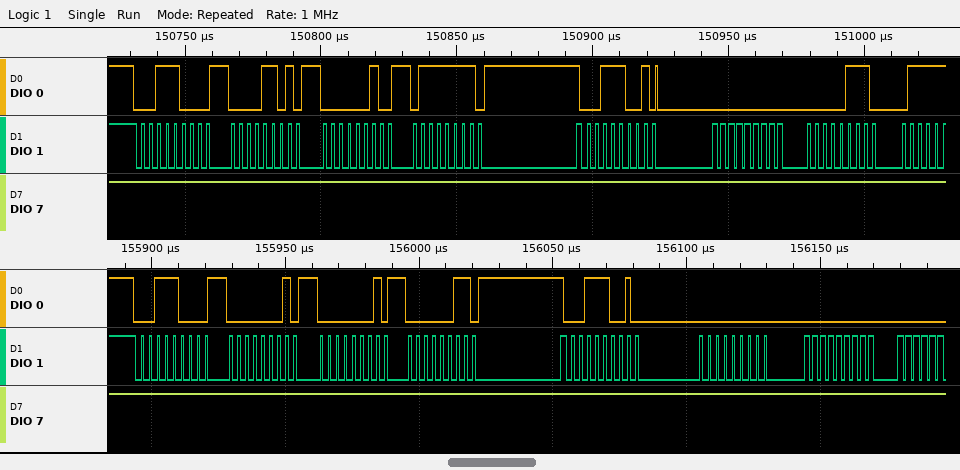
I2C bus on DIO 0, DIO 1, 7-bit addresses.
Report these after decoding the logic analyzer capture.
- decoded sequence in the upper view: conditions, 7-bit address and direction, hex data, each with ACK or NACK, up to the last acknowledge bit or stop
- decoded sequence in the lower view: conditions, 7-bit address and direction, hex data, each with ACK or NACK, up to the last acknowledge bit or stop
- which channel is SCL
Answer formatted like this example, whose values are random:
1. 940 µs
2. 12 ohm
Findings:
1. start, address 1C write ACK, 0D ACK, 02 ACK, 7F ACK, repeated start, address 1C read ACK, 00 ACK, 07 ACK
2. start, address 1C write ACK, 01 ACK, 01 ACK, 03 ACK, repeated start, address 1C read ACK, 00 ACK, 00 ACK
3. DIO 1
